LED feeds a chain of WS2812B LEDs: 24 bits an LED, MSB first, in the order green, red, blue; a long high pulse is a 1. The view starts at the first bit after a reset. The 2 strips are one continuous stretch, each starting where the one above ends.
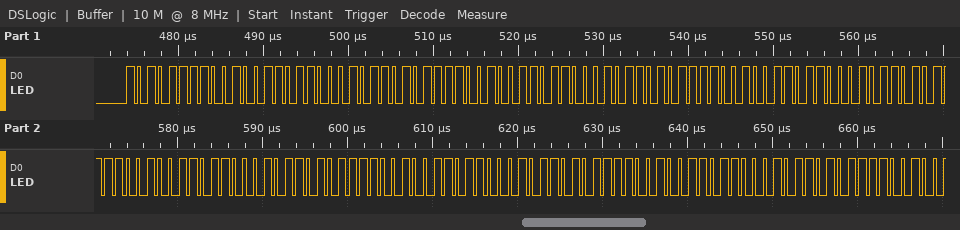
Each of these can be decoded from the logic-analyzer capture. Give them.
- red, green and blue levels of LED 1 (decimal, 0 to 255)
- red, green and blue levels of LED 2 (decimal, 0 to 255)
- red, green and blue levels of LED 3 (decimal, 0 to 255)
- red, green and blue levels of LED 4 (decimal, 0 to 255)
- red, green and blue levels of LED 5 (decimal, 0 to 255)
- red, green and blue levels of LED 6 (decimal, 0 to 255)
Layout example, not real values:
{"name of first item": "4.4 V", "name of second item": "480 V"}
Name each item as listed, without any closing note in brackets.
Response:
{"red, green and blue levels of LED 1": "38, 175, 197", "red, green and blue levels of LED 2": "38, 175, 197", "red, green and blue levels of LED 3": "38, 175, 197", "red, green and blue levels of LED 4": "38, 175, 197", "red, green and blue levels of LED 5": "38, 175, 197", "red, green and blue levels of LED 6": "38, 175, 197"}
